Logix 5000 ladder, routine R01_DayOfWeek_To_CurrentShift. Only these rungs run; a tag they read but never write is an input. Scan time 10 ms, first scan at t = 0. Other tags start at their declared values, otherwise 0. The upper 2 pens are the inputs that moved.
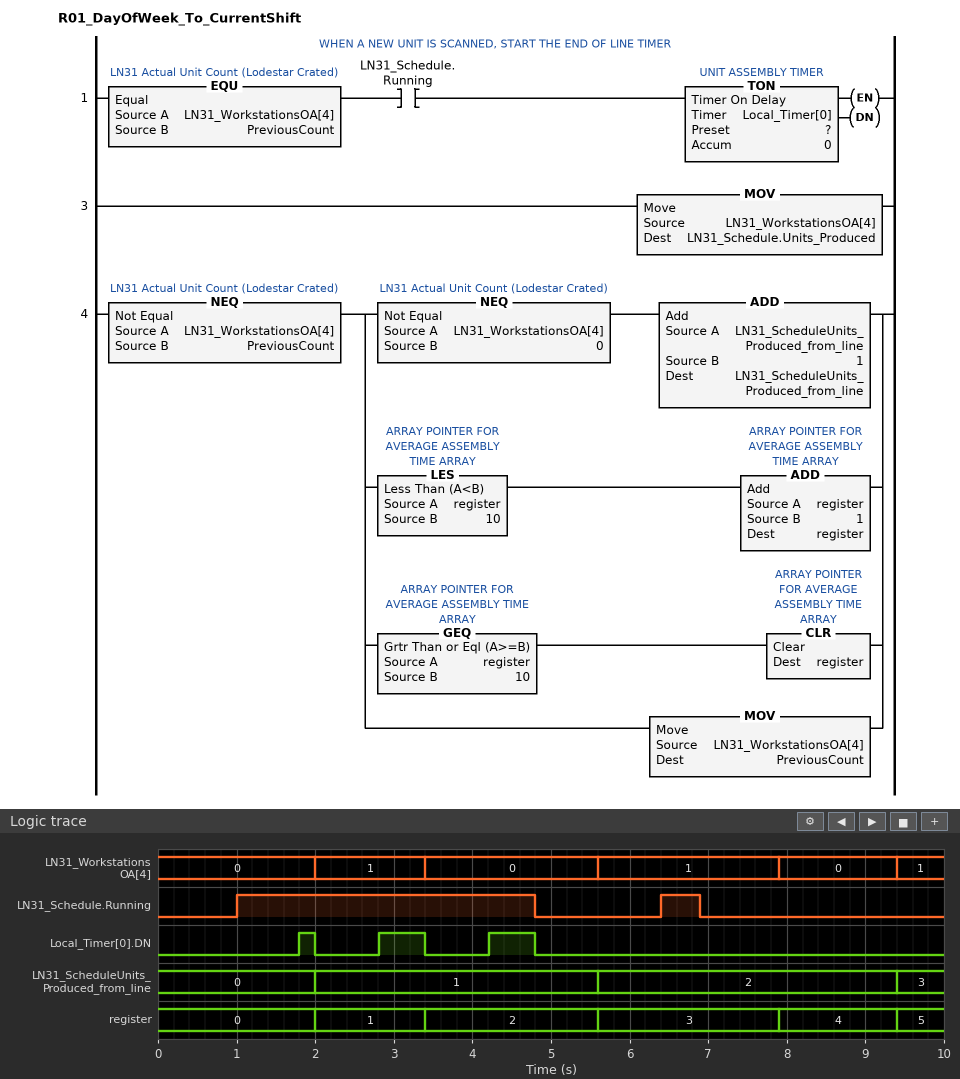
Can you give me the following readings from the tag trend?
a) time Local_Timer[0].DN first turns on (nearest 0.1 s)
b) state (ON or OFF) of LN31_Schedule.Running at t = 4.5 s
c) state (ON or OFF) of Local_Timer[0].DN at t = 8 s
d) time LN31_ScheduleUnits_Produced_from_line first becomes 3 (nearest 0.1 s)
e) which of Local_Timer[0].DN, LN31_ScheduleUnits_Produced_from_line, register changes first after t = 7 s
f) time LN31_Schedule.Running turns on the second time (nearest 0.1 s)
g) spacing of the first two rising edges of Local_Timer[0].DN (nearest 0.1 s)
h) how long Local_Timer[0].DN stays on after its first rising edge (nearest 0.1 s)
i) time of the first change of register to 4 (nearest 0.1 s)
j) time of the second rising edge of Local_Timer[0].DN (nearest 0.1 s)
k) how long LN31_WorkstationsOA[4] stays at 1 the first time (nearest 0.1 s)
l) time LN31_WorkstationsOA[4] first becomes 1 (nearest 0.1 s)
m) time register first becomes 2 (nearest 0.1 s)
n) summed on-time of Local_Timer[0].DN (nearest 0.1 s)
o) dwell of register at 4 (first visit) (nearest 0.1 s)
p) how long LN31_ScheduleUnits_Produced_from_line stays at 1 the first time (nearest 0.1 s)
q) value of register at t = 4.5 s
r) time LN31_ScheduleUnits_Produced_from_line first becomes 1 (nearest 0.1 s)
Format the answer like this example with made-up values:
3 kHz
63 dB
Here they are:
1.8 s
ON
OFF
9.4 s
register
6.4 s
1.0 s
0.2 s
7.9 s
2.8 s
1.4 s
2.0 s
3.4 s
1.4 s
1.5 s
3.6 s
2
2.0 s
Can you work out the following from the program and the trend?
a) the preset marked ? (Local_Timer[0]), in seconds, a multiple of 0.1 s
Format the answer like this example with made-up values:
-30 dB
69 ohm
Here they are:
0.8 s
